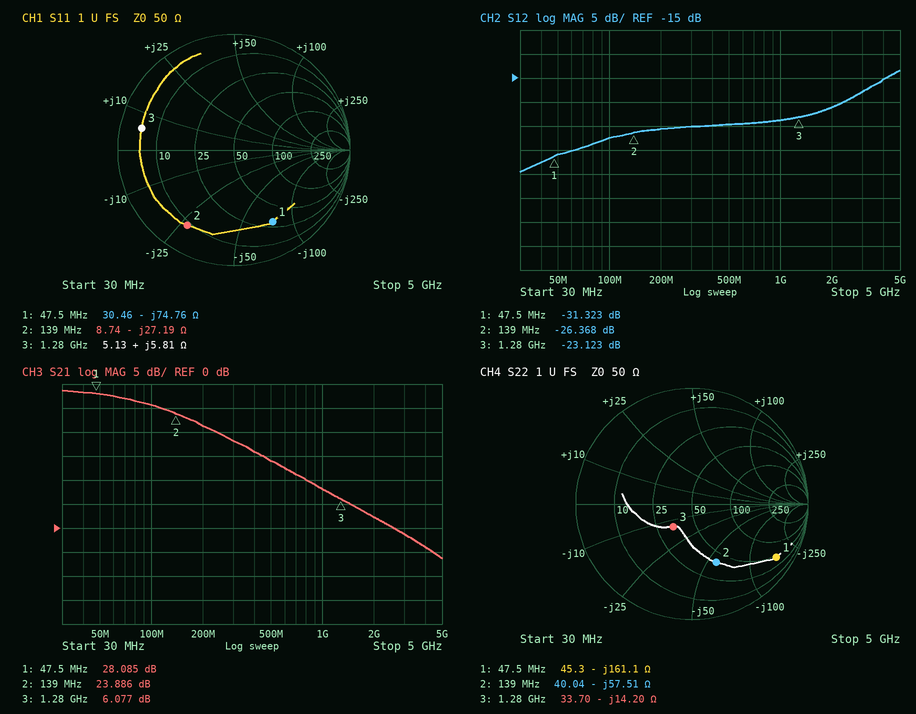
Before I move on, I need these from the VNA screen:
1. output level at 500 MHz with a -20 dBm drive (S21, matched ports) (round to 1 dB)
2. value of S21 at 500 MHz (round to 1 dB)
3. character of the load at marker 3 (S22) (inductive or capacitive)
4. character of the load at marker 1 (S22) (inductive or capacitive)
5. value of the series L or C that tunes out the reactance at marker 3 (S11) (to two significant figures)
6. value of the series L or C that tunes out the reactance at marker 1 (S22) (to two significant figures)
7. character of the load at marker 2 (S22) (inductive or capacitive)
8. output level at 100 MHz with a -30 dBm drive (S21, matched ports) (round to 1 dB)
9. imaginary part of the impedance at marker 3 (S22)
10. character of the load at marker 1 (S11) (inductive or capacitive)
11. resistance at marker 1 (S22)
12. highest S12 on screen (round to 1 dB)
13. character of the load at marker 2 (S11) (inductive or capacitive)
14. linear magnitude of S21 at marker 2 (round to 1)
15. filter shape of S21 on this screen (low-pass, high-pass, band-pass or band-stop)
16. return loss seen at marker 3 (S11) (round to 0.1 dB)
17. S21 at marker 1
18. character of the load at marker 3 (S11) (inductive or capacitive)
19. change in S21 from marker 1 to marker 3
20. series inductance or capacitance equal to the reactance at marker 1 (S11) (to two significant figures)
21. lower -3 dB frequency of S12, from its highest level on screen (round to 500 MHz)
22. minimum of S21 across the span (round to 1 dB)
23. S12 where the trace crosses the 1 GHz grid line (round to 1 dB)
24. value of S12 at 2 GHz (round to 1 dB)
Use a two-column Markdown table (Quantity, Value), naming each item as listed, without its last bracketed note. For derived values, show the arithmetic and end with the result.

| Quantity | Value |
|---|---|
| output level at 500 MHz with a -20 dBm drive (S21, matched ports) | -20 dBm + (14 dB) = -6 dBm |
| value of S21 at 500 MHz | 14 dB |
| character of the load at marker 3 (S22) | capacitive |
| character of the load at marker 1 (S22) | capacitive |
| value of the series L or C that tunes out the reactance at marker 3 (S11) | C = 1/(2π × 1.28 GHz × 5.81 Ω) ≈ 21 pF |
| value of the series L or C that tunes out the reactance at marker 1 (S22) | L = 161.1 Ω/(2π × 47.5 MHz) ≈ 540 nH |
| character of the load at marker 2 (S22) | capacitive |
| output level at 100 MHz with a -30 dBm drive (S21, matched ports) | -30 dBm + (26 dB) = -4 dBm |
| imaginary part of the impedance at marker 3 | -14.20 Ω |
| character of the load at marker 1 (S11) | capacitive |
| resistance at marker 1 | 45.3 Ω |
| highest S12 on screen | -13 dB |
| character of the load at marker 2 (S11) | capacitive |
| linear magnitude of S21 at marker 2 | 10^(23.886/20) ≈ 16 |
| filter shape of S21 on this screen | low-pass |
| return loss seen at marker 3 (S11) | 1.8 dB |
| S21 at marker 1 | 28.085 dB |
| character of the load at marker 3 (S11) | inductive |
| change in S21 from marker 1 to marker 3 | 6.077 − (28.085) = -22.008 dB |
| series inductance or capacitance equal to the reactance at marker 1 (S11) | C = 1/(2π × 47.5 MHz × 74.76 Ω) ≈ 45 pF |
| lower -3 dB frequency of S12, from its highest level on screen | 3.5 GHz |
| minimum of S21 across the span | -6 dB |
| S12 where the trace crosses the 1 GHz grid line | -24 dB |
| value of S12 at 2 GHz | -21 dB |
